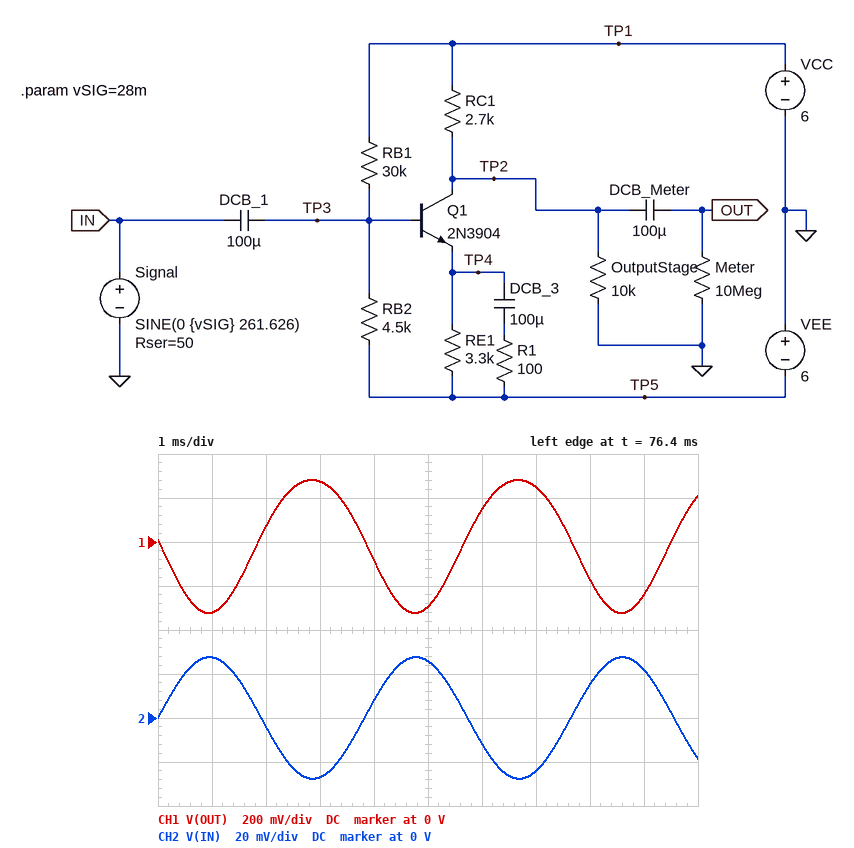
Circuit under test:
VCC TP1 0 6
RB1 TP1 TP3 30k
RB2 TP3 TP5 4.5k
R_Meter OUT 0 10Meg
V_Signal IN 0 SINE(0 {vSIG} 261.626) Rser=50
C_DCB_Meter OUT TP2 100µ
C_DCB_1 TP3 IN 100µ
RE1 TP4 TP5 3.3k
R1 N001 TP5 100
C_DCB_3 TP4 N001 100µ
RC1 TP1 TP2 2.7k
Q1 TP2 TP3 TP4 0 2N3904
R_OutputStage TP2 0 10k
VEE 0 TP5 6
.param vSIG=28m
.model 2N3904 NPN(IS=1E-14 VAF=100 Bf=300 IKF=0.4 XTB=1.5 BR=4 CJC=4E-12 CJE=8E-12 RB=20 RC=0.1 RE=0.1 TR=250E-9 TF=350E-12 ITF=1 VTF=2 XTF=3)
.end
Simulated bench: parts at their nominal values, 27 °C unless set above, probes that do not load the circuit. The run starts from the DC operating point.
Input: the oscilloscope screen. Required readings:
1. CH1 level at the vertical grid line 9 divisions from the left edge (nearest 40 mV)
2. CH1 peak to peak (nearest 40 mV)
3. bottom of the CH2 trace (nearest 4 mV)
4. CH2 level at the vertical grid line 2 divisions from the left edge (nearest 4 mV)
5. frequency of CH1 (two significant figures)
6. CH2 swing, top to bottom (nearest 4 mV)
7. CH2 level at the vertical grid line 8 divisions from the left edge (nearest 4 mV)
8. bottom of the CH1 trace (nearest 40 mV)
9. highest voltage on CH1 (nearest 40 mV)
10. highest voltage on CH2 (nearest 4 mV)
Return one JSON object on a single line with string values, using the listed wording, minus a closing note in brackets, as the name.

{"CH1 level at the vertical grid line 9 divisions from the left edge": "-240 mV", "CH1 peak to peak": "600 mV", "bottom of the CH2 trace": "-28 mV", "CH2 level at the vertical grid line 2 divisions from the left edge": "-4 mV", "frequency of CH1": "260 Hz", "CH2 swing, top to bottom": "56 mV", "CH2 level at the vertical grid line 8 divisions from the left edge": "16 mV", "bottom of the CH1 trace": "-320 mV", "highest voltage on CH1": "280 mV", "highest voltage on CH2": "28 mV"}
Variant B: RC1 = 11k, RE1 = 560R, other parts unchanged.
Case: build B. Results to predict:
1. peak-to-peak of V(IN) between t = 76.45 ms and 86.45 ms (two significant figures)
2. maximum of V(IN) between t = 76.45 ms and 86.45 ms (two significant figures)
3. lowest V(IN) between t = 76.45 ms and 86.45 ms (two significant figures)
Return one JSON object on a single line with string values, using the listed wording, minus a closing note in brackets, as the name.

{"peak-to-peak of V(IN) between t = 76.45 ms and 86.45 ms": "50 mV", "maximum of V(IN) between t = 76.45 ms and 86.45 ms": "23 mV", "lowest V(IN) between t = 76.45 ms and 86.45 ms": "-27 mV"}
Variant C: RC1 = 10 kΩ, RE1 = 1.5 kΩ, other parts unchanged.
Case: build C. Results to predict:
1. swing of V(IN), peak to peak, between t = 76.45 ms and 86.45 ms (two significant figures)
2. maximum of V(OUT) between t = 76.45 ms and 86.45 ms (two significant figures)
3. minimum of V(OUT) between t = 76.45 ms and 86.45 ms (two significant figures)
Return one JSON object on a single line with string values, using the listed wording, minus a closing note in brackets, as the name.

{"swing of V(IN), peak to peak, between t = 76.45 ms and 86.45 ms": "55 mV", "maximum of V(OUT) between t = 76.45 ms and 86.45 ms": "960 mV", "minimum of V(OUT) between t = 76.45 ms and 86.45 ms": "-1.0 V"}
